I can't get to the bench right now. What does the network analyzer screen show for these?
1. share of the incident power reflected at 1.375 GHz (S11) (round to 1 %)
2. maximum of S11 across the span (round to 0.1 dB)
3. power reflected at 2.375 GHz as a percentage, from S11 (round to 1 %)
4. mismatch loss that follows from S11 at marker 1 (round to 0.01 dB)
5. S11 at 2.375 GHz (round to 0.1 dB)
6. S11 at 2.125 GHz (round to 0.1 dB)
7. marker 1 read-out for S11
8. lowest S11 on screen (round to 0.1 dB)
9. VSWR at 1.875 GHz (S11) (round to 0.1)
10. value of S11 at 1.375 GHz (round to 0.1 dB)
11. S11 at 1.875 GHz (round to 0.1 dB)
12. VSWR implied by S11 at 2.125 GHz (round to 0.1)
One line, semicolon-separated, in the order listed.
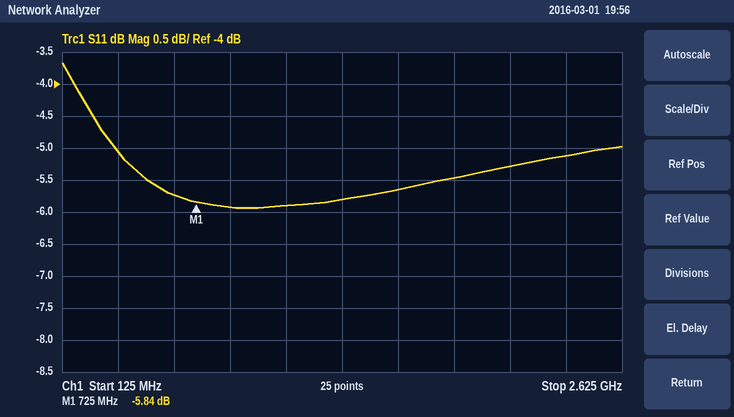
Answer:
26 %; -3.7 dB; 31 %; 1.31 dB; -5.1 dB; -5.3 dB; -5.84 dB; -5.9 dB; 3.3; -5.8 dB; -5.5 dB; 3.4
